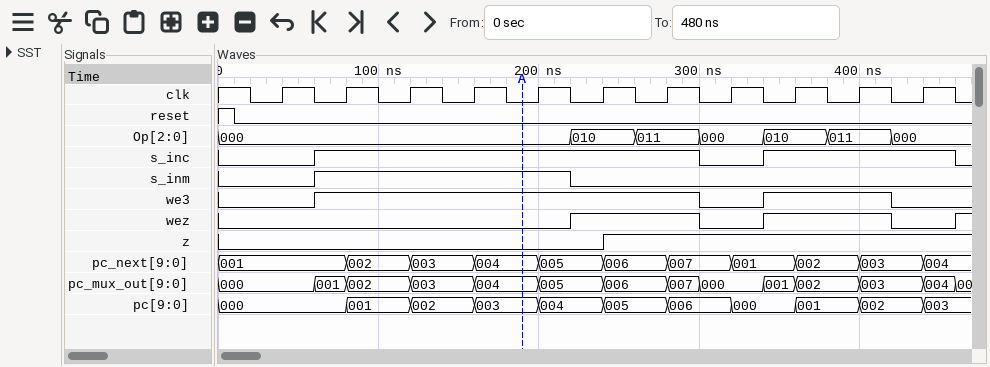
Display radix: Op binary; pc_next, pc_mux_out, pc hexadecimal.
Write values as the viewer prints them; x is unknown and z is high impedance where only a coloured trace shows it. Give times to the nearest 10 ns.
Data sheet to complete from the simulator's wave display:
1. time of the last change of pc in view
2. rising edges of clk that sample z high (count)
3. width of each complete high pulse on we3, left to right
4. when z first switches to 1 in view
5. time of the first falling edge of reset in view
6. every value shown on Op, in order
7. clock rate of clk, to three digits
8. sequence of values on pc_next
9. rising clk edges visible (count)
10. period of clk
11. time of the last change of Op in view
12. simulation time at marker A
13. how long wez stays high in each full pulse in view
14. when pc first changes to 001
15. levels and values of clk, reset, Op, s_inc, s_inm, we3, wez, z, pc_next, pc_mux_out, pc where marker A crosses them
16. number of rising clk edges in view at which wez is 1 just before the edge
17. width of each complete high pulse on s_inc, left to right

440 ns
5
240 ns, 80 ns
240 ns
10 ns
000, 010, 011, 000, 010, 011, 000
25.0 MHz
001, 002, 003, 004, 005, 006, 007, 001, 002, 003, 004
11
40 ns
420 ns
190 ns
80 ns, 80 ns
80 ns
clk=0, reset=0, Op=000, s_inc=1, s_inm=1, we3=1, wez=0, z=0, pc_next=004, pc_mux_out=004, pc=003
4
240 ns, 120 ns
